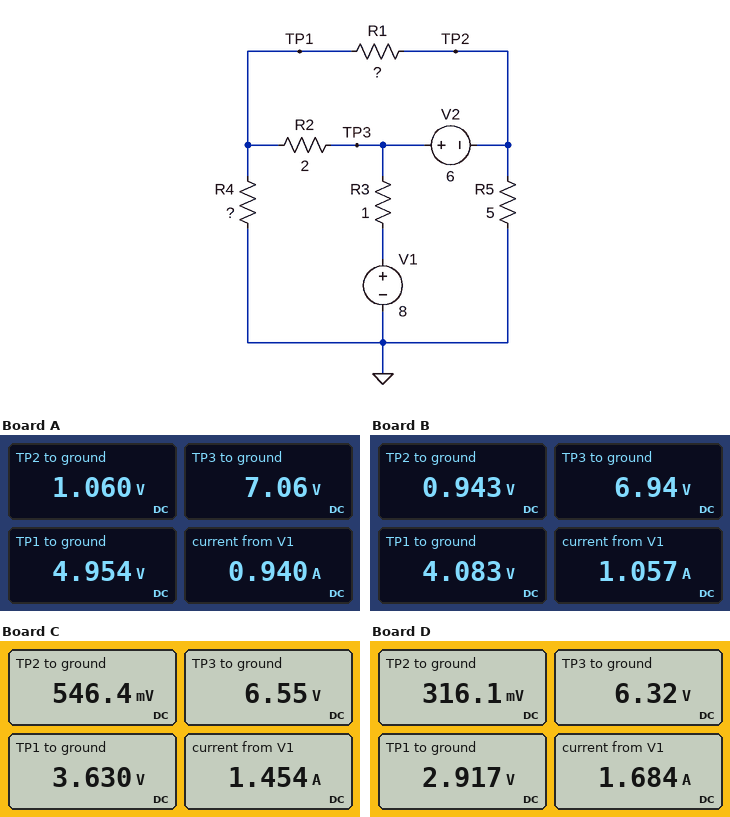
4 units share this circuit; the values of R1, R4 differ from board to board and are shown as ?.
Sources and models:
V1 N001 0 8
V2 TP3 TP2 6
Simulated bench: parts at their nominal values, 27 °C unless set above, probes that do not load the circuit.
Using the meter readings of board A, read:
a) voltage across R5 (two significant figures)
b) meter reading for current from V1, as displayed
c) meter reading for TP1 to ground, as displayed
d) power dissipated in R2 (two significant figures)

1.1 V
0.940 A
4.954 V
2.2 W
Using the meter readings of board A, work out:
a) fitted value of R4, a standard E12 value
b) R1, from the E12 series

6.8 Ω
12 Ω
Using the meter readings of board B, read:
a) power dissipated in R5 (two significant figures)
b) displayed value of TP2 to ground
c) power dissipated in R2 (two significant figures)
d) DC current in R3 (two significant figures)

180 mW
0.943 V
4.1 W
1.1 A
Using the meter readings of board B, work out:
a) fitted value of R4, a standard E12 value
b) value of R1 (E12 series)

4.7 Ω
5.6 Ω
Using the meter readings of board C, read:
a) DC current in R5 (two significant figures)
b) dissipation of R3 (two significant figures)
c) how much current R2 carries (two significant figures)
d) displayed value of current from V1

110 mA
2.1 W
1.5 A
1.454 A
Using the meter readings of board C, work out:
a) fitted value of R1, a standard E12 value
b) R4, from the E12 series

27 Ω
2.7 Ω
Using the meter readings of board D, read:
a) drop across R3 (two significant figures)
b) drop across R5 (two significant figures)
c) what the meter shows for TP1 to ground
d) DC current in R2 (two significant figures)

1.7 V
320 mV
2.917 V
1.7 A
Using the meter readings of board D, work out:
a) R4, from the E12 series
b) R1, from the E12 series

1.8 Ω
33 Ω
